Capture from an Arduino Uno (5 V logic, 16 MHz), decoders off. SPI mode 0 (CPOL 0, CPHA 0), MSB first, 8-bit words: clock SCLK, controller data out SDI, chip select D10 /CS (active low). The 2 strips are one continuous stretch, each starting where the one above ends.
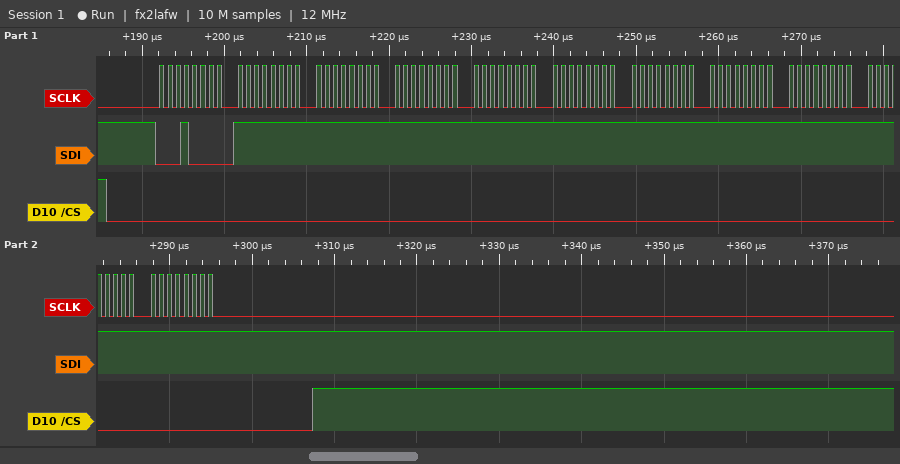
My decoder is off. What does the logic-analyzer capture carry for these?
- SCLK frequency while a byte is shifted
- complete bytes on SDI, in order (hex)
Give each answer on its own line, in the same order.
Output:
1 MHz
10 FF FF FF FF FF FF FF FF FF FF
